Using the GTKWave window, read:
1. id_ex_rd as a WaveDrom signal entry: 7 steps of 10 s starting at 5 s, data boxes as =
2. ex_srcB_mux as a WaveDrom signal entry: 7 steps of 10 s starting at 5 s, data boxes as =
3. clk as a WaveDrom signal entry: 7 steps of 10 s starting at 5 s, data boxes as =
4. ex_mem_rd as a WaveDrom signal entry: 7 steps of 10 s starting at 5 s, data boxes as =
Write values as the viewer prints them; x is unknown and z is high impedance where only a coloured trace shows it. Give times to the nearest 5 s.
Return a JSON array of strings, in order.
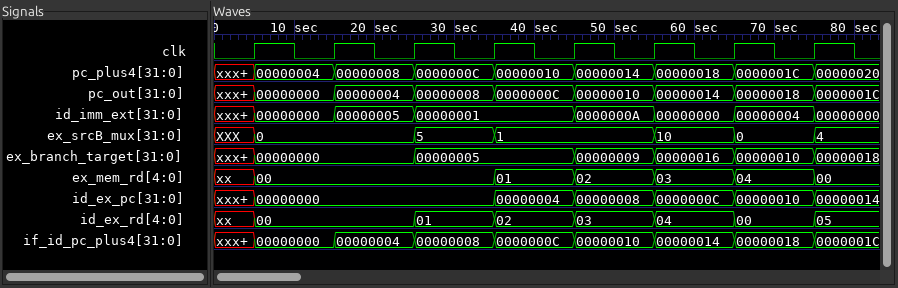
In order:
["{name: 'id_ex_rd', wave: '=.=====', data: '00 01 02 03 04 00'}", "{name: 'ex_srcB_mux', wave: '=.==.==', data: '0 5 1 10 0'}", "{name: 'clk', wave: 'p......'}", "{name: 'ex_mem_rd', wave: '=..====', data: '00 01 02 03 04'}"]
